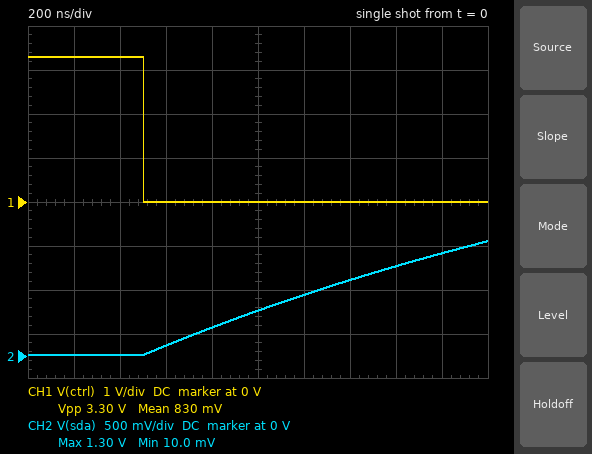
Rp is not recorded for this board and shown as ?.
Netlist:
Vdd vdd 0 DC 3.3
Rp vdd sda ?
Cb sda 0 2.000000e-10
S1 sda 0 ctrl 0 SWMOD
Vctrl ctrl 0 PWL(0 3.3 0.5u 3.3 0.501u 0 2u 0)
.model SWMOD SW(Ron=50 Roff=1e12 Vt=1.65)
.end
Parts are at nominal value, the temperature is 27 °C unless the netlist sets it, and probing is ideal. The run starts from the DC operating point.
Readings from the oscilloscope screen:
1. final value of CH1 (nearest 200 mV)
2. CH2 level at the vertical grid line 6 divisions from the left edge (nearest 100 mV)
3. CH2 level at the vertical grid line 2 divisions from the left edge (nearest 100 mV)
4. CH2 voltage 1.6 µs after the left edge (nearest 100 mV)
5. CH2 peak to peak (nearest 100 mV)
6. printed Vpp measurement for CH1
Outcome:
0 V
700 mV
0 V
1.0 V
1.3 V
3.30 V
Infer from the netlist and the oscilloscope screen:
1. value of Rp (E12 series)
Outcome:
15 kΩ
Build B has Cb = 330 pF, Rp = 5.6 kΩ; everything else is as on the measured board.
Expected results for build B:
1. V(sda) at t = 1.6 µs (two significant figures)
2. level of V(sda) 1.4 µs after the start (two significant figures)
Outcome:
1.5 V
1.3 V
